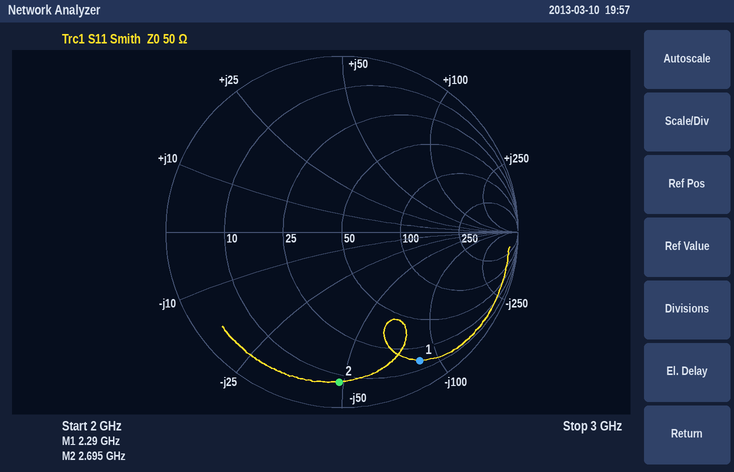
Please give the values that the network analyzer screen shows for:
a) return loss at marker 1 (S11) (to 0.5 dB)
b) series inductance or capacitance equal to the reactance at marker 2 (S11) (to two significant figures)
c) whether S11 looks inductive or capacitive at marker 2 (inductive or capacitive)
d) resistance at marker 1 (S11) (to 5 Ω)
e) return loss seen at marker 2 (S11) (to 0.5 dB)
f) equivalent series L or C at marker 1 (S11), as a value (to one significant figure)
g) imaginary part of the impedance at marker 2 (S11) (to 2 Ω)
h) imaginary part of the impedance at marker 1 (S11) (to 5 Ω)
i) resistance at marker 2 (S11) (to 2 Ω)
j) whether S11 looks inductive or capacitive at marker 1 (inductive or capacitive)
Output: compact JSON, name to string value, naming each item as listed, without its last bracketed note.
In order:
{"return loss at marker 1 (S11)": "1.5 dB", "series inductance or capacitance equal to the reactance at marker 2 (S11)": "1.2 pF", "whether S11 looks inductive or capacitive at marker 2": "capacitive", "resistance at marker 1 (S11)": "15 Ω", "return loss seen at marker 2 (S11)": "1.5 dB", "equivalent series L or C at marker 1 (S11), as a value": "800 fF", "imaginary part of the impedance at marker 2 (S11)": "-48 Ω", "imaginary part of the impedance at marker 1 (S11)": "-85 Ω", "resistance at marker 2 (S11)": "8 Ω", "whether S11 looks inductive or capacitive at marker 1": "capacitive"}
